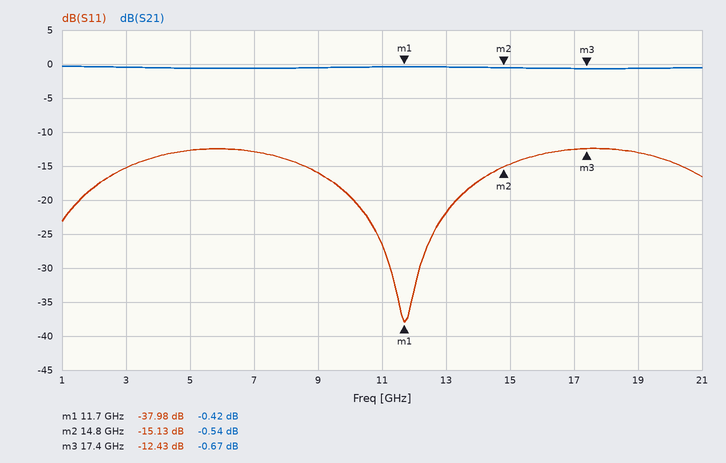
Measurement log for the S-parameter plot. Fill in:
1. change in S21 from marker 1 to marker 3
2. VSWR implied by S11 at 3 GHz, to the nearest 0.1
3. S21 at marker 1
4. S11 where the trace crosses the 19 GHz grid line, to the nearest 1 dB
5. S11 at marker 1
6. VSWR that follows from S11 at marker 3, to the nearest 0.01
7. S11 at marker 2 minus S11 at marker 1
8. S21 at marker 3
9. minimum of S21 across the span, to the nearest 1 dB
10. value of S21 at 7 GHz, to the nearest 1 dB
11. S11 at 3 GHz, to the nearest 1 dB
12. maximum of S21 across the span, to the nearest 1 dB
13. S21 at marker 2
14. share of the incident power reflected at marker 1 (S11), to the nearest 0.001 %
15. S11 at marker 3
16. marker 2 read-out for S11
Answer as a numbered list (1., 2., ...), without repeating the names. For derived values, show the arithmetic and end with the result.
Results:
1. -0.67 − (-0.42) = -0.25 dB
2. |Γ| = 10^(-15/20) = 0.1778; VSWR = (1 + 0.1778)/(1 − 0.1778) ≈ 1.4
3. -0.42 dB
4. -13 dB
5. -37.98 dB
6. (1 + 0.2391)/(1 − 0.2391) ≈ 1.63
7. -15.13 − (-37.98) = 22.85 dB
8. -0.67 dB
9. -1 dB
10. -1 dB
11. -15 dB
12. 0 dB
13. -0.54 dB
14. 10^(-37.98/10) ≈ 0.016 %
15. -12.43 dB
16. -15.13 dB
